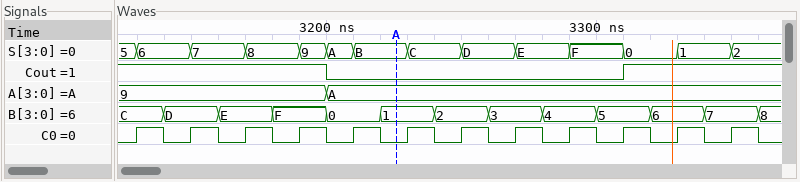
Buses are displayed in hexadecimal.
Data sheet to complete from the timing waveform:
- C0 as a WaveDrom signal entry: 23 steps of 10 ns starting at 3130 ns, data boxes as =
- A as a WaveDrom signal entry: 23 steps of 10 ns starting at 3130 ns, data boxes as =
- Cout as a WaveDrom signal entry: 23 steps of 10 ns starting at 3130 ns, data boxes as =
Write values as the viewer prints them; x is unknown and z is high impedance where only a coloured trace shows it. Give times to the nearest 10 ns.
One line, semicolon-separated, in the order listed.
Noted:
{name: 'C0', wave: '10101010101010101010101'}; {name: 'A', wave: '=......=...............', data: '9 A'}; {name: 'Cout', wave: '1......0..........1....'}
